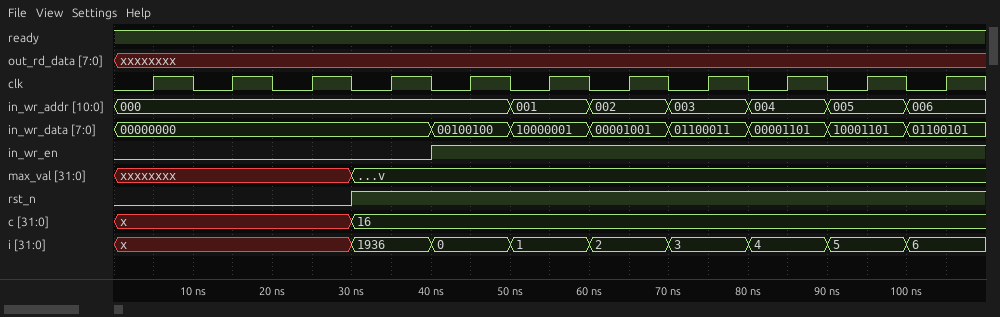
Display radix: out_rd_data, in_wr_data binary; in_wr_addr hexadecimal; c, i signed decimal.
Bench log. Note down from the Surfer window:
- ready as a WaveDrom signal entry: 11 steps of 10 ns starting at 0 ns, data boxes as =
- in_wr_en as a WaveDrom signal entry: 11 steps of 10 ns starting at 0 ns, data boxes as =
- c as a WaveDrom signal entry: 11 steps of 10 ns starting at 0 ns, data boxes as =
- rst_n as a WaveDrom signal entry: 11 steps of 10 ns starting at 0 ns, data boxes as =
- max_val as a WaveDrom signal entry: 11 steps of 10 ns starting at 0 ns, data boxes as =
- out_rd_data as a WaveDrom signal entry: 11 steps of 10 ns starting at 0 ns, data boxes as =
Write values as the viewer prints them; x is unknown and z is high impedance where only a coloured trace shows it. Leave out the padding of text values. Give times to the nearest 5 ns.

{name: 'ready', wave: '1..........'}
{name: 'in_wr_en', wave: '0...1......'}
{name: 'c', wave: 'x..=.......', data: '16'}
{name: 'rst_n', wave: '0..1.......'}
{name: 'max_val', wave: 'x..=.......', data: 'v'}
{name: 'out_rd_data', wave: 'x..........'}
